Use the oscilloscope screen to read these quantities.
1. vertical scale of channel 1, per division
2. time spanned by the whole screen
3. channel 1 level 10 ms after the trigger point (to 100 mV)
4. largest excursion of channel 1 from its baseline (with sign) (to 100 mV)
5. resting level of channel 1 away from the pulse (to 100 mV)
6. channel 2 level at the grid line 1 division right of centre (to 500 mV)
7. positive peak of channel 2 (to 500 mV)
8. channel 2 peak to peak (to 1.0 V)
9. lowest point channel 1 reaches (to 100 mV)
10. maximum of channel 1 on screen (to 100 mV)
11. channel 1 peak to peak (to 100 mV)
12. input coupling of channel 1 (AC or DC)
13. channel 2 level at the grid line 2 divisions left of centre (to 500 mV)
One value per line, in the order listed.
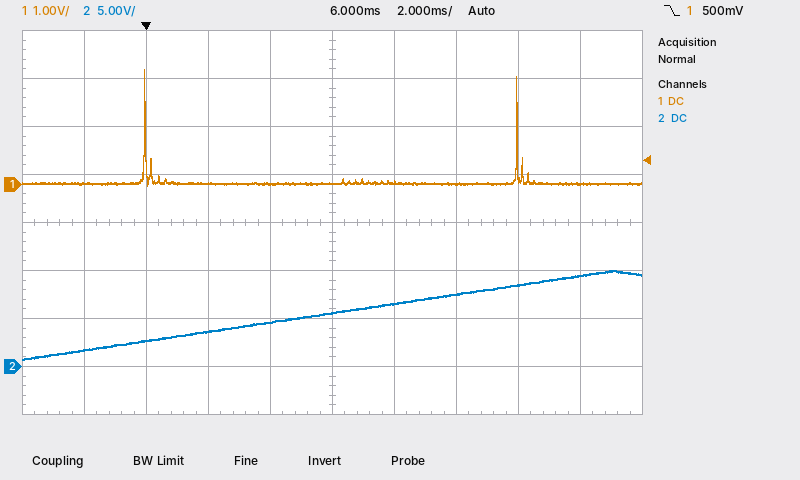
1 V
20 ms
0.0 V
+2.4 V
0.0 V
6.5 V
10.0 V
9.0 V
0.0 V
2.4 V
2.4 V
DC
3.5 V
